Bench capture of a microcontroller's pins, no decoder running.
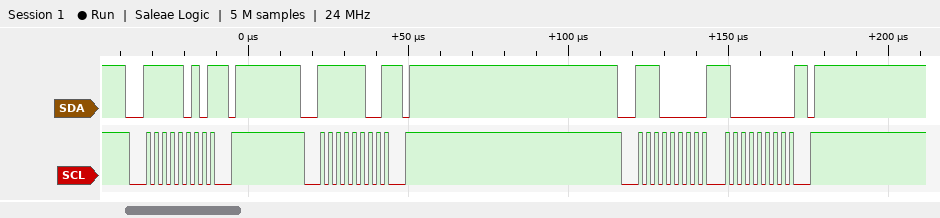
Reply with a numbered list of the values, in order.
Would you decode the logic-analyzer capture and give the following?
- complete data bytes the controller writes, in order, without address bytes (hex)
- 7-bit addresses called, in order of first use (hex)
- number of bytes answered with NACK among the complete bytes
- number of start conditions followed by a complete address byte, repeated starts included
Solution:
1. 80
2. 0x7D 0x7E 0x70
3. 2
4. 3
